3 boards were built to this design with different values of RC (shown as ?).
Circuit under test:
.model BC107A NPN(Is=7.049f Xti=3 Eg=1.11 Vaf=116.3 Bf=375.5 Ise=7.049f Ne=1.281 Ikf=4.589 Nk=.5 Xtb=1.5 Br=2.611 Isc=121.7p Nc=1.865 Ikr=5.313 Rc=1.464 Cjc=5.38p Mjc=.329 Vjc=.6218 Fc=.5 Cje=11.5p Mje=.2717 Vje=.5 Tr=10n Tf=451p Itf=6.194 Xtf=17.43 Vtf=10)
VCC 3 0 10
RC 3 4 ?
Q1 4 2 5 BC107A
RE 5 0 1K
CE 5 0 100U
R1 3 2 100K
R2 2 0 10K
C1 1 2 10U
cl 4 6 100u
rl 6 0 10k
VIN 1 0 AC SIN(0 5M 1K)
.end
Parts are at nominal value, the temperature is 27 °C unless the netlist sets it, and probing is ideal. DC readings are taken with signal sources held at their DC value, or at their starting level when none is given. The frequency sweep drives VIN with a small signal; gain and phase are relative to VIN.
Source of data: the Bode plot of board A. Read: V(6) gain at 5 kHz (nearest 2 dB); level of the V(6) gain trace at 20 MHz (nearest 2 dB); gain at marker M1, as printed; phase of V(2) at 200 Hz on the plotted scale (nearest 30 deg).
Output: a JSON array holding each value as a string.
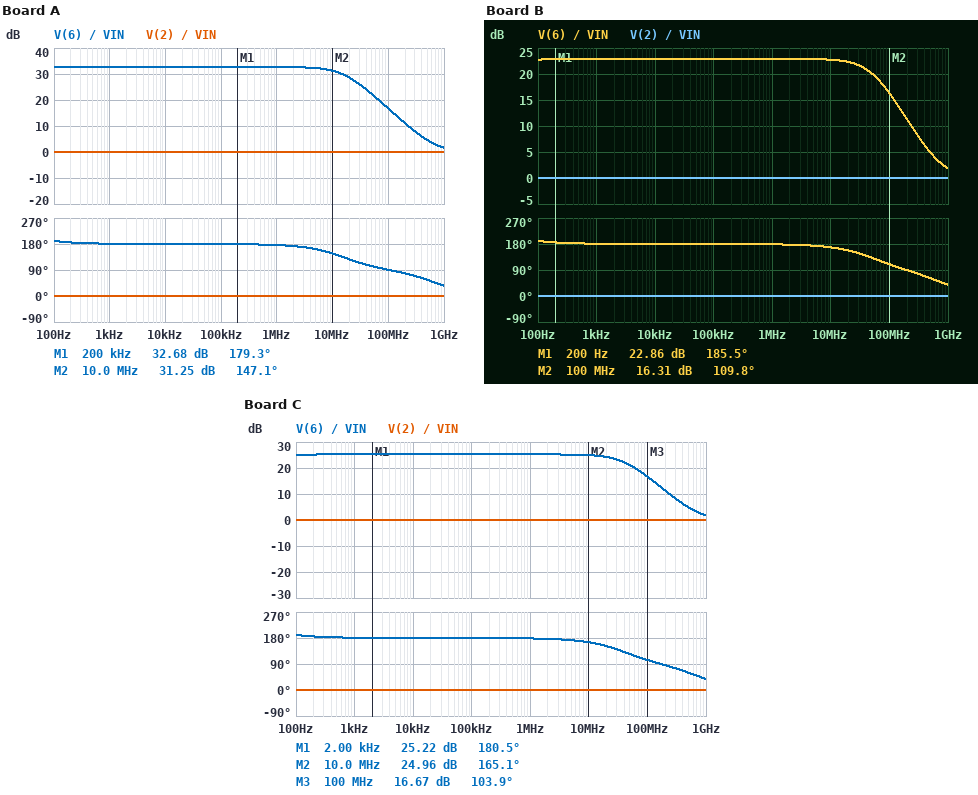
["32 dB", "28 dB", "32.68 dB", "0 deg"]
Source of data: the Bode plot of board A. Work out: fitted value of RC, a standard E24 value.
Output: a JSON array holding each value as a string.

["7.5 kΩ"]
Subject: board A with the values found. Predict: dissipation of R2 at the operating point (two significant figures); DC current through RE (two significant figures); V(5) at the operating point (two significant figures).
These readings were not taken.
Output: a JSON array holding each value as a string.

["80 µW", "260 µA", "260 mV"]
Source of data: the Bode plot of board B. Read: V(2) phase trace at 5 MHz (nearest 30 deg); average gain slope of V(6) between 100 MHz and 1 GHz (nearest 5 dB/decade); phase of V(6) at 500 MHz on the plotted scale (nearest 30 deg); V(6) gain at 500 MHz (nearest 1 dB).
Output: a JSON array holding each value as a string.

["0 deg", "-15 dB/decade", "60 deg", "5 dB"]
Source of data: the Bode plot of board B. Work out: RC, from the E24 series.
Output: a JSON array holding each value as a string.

["1.6 kΩ"]
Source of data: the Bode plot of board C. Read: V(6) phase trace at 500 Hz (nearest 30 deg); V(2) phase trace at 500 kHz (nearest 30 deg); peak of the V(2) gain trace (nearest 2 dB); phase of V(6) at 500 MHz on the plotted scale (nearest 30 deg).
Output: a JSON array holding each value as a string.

["180 deg", "0 deg", "0 dB", "60 deg"]
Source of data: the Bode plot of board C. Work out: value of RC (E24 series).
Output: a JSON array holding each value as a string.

["2.2 kΩ"]
